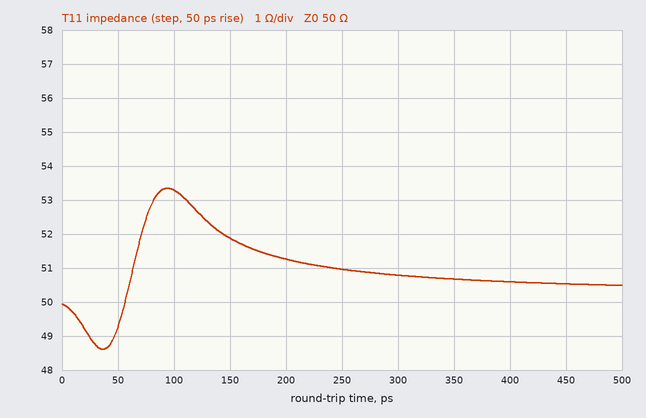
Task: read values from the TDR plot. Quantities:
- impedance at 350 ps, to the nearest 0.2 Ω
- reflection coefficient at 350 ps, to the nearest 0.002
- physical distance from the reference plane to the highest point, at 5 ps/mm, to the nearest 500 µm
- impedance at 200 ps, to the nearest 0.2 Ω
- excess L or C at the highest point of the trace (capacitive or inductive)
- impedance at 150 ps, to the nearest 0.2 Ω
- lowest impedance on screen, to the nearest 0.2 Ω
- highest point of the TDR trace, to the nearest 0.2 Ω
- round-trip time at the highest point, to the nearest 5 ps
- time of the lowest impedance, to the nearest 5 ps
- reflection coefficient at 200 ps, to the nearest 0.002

50.6 Ω
+0.006
9.5 mm
51.2 Ω
inductive
51.8 Ω
48.6 Ω
53.4 Ω
95 ps
35 ps
+0.012
